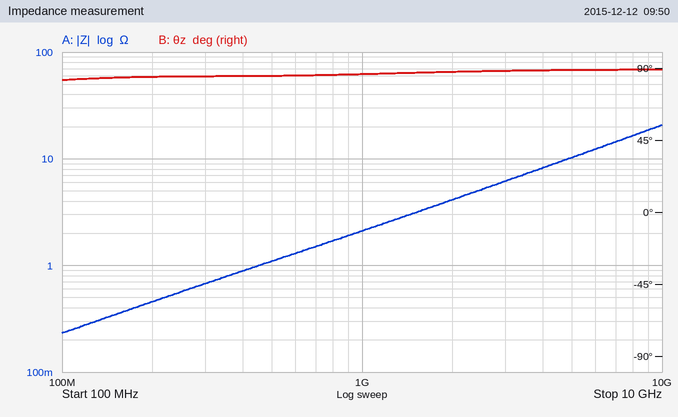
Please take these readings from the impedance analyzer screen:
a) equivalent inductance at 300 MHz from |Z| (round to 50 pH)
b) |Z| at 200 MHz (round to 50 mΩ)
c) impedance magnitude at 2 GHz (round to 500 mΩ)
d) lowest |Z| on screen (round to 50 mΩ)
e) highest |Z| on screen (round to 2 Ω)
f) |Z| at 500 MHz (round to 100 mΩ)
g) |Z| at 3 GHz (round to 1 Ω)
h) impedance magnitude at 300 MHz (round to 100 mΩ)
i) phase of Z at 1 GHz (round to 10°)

350 pH
450 mΩ
4.0 Ω
250 mΩ
20 Ω
1.1 Ω
6 Ω
700 mΩ
90°
